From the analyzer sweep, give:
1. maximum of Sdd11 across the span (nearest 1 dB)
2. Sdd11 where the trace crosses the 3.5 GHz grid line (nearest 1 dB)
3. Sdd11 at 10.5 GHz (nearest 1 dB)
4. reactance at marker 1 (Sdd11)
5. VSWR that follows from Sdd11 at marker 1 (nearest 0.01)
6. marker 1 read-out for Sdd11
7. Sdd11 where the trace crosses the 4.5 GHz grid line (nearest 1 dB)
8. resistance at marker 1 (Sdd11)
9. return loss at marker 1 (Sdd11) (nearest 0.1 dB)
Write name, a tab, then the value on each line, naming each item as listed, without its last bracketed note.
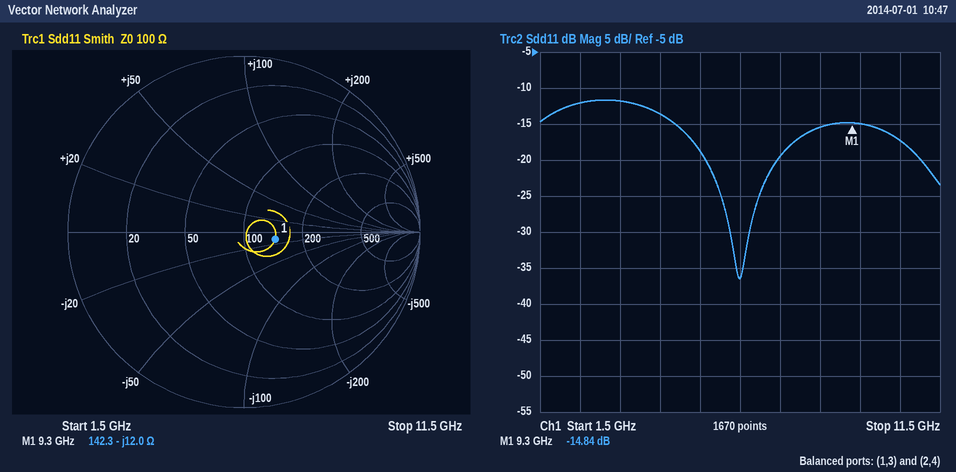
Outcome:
maximum of Sdd11 across the span	-12 dB
Sdd11 where the trace crosses the 3.5 GHz grid line	-12 dB
Sdd11 at 10.5 GHz	-17 dB
reactance at marker 1	-12.0 Ω
VSWR that follows from Sdd11 at marker 1	1.44
marker 1 read-out for Sdd11	-14.84 dB
Sdd11 where the trace crosses the 4.5 GHz grid line	-14 dB
resistance at marker 1	142.3 Ω
return loss at marker 1 (Sdd11)	14.8 dB
